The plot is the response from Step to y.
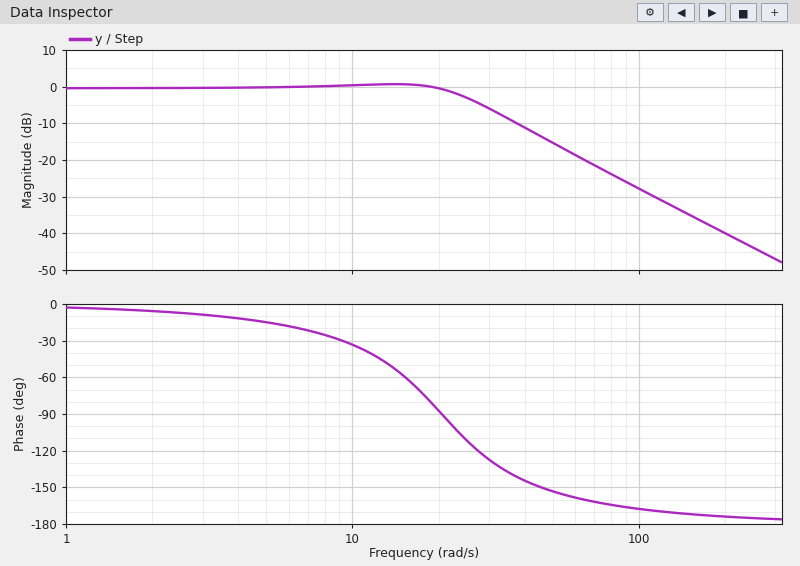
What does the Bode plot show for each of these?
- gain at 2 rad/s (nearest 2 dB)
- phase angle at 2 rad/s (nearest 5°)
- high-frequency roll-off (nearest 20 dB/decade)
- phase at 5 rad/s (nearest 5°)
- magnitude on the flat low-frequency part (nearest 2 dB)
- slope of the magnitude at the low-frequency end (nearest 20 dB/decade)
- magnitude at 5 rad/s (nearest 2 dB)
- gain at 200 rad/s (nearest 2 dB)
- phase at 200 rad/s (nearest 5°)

0 dB
-5°
-40 dB/decade
-15°
0 dB
0 dB/decade
0 dB
-40 dB
-175°
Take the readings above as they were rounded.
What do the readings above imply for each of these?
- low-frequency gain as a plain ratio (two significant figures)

1.0
